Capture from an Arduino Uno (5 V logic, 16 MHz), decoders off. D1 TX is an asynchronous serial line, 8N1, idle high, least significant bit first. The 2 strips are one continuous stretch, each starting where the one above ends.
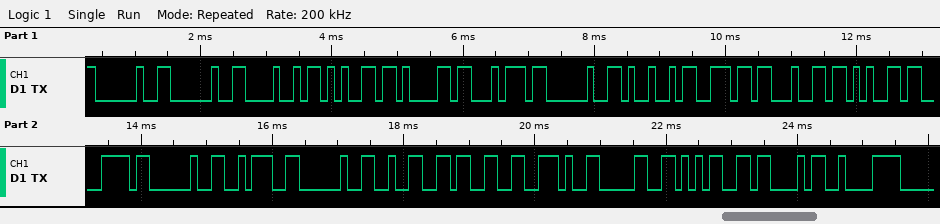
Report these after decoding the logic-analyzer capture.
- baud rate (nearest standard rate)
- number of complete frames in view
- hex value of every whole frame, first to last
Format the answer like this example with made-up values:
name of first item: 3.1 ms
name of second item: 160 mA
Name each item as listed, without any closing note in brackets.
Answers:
baud rate: 9600 baud
number of complete frames in view: 22
hex value of every whole frame, first to last: 20 20 48 65 61 74 20 49 6E 64 65 78 20 3A 20 32 33 2E 30 35 43 C2
